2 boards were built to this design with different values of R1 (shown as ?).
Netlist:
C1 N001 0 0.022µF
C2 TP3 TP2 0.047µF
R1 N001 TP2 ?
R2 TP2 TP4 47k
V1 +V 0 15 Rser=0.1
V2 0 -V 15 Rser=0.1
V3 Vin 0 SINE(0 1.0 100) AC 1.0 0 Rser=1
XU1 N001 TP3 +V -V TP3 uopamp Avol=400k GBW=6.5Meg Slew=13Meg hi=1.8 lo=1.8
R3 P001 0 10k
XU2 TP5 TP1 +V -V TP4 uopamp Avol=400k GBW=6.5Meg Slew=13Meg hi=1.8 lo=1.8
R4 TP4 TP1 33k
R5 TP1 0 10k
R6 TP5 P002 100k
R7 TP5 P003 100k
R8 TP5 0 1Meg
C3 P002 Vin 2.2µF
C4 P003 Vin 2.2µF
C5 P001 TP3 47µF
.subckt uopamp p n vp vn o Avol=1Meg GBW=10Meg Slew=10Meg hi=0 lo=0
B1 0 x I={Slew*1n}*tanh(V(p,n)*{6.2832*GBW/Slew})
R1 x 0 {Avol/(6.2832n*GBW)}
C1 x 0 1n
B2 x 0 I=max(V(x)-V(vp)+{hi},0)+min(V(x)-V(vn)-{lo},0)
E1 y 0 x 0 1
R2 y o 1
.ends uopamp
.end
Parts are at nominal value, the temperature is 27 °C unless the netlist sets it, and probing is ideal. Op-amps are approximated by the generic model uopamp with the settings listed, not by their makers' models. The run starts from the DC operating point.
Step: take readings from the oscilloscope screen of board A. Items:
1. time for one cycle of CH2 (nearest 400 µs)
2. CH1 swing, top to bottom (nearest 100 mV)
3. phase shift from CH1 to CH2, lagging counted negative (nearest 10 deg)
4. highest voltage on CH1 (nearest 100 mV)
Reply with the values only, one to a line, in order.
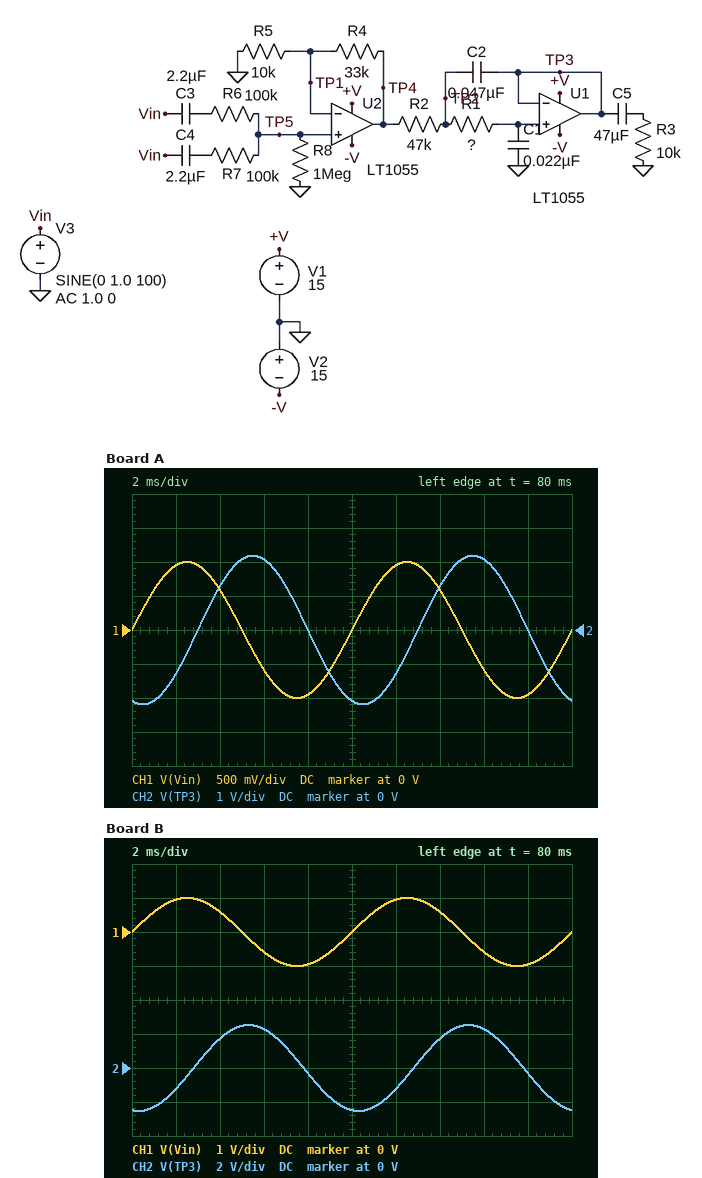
10.0 ms
2.0 V
-110 deg
1.0 V
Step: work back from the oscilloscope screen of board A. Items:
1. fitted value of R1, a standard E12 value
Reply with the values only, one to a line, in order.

82 kΩ
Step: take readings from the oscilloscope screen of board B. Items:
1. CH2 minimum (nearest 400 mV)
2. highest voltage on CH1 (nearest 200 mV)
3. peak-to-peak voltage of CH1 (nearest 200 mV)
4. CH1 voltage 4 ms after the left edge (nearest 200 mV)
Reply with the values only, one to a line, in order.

-2.4 V
1.0 V
2.0 V
600 mV
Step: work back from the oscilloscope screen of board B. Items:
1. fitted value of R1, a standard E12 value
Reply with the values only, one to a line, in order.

68 kΩ
